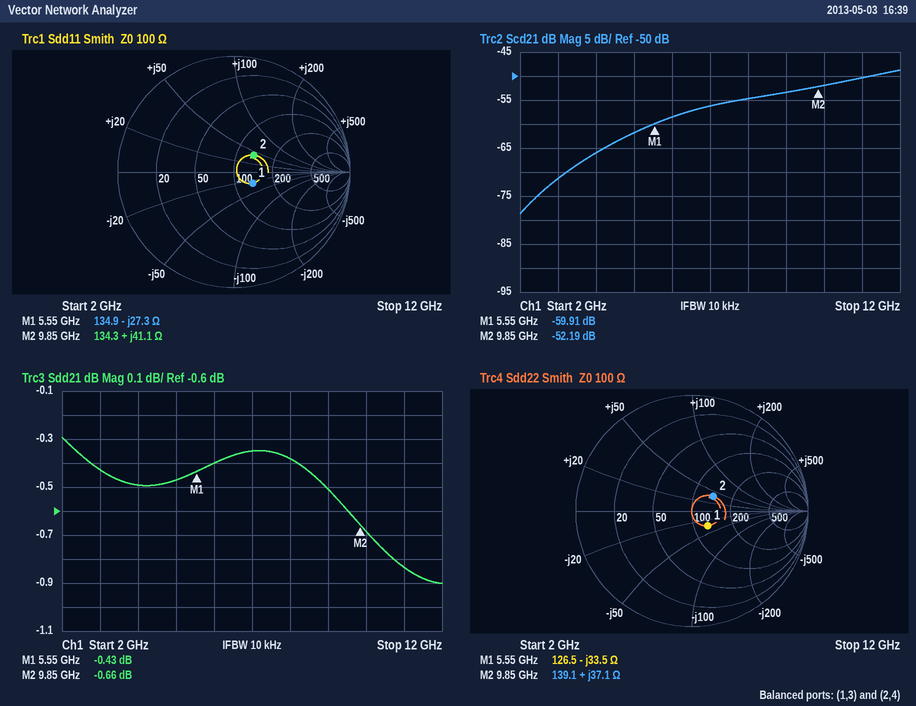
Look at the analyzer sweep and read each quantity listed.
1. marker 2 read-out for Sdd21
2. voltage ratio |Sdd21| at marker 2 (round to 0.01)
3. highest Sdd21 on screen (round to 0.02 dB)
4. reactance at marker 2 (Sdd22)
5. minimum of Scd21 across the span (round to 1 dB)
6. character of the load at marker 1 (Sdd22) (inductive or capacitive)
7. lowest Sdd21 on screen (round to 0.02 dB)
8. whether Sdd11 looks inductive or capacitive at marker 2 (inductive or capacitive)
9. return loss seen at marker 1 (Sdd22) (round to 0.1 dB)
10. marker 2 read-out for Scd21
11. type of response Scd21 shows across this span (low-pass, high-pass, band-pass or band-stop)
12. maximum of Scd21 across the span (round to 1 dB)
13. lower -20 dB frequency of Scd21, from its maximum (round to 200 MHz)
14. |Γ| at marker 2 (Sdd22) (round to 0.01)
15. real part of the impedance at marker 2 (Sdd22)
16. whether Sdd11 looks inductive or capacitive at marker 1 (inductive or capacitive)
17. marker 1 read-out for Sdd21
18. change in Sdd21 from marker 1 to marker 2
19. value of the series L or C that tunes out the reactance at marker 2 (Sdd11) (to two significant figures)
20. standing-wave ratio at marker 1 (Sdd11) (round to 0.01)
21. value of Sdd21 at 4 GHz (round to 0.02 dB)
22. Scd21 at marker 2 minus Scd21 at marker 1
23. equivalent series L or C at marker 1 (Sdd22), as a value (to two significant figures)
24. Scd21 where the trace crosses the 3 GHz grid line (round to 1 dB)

-0.66 dB
0.93
-0.30 dB
+37.1 Ω
-79 dB
capacitive
-0.90 dB
inductive
14.6 dB
-52.19 dB
high-pass
-49 dB
3.4 GHz
0.22
139.1 Ω
capacitive
-0.43 dB
-0.23 dB
390 fF
1.46
-0.50 dB
7.72 dB
860 fF
-71 dB
